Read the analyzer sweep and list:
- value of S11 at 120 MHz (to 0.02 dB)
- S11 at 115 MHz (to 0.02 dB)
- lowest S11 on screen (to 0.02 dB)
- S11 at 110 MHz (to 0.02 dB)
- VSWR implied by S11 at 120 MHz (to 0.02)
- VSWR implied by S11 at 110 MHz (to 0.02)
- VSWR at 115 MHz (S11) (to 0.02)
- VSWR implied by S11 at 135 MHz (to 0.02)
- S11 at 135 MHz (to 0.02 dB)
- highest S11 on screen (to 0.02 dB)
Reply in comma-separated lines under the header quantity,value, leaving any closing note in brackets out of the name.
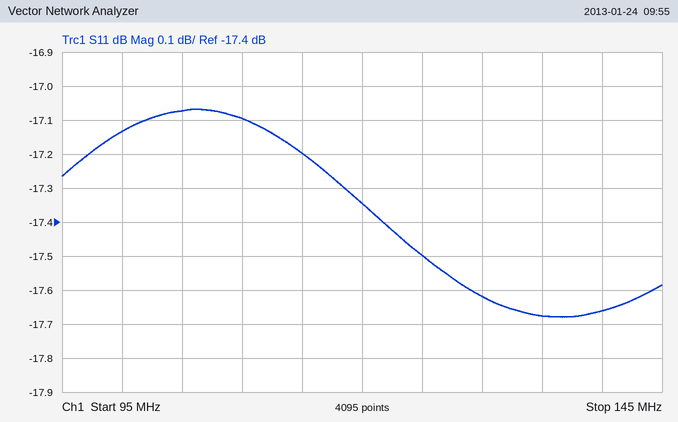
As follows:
quantity,value
value of S11 at 120 MHz,-17.34 dB
S11 at 115 MHz,-17.20 dB
lowest S11 on screen,-17.68 dB
S11 at 110 MHz,-17.10 dB
VSWR implied by S11 at 120 MHz,1.32
VSWR implied by S11 at 110 MHz,1.32
VSWR at 115 MHz (S11),1.32
VSWR implied by S11 at 135 MHz,1.30
S11 at 135 MHz,-17.68 dB
highest S11 on screen,-17.06 dB
